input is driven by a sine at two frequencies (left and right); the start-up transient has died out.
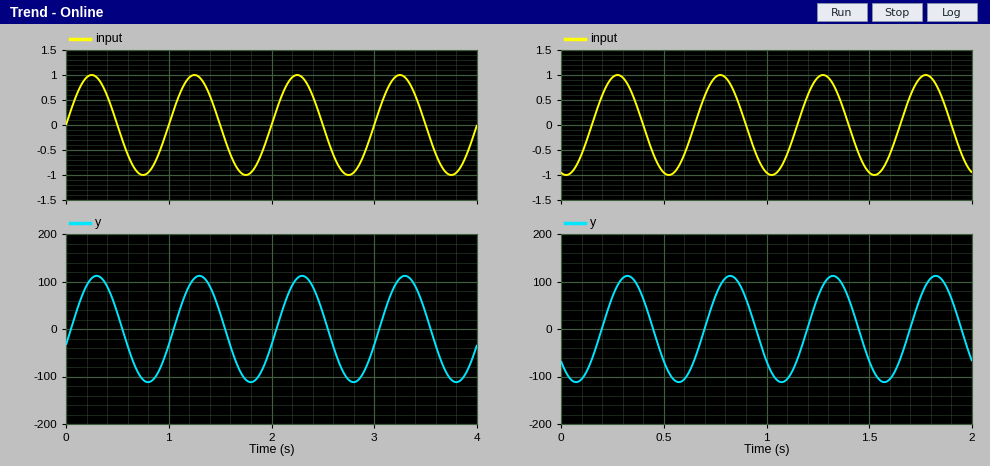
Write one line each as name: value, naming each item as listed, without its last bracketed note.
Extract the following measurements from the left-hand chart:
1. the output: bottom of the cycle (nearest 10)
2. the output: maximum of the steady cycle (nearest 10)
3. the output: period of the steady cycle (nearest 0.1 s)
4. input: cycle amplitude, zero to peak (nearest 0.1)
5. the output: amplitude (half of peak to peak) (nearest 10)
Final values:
the output: bottom of the cycle: -110
the output: maximum of the steady cycle: 110
the output: period of the steady cycle: 1.0 s
input: cycle amplitude, zero to peak: 1.0
the output: amplitude (half of peak to peak): 110
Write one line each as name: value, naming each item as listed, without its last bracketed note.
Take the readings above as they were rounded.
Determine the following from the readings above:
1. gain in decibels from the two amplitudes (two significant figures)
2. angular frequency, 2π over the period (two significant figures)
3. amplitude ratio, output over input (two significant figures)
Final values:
gain in decibels from the two amplitudes: 41 dB
angular frequency, 2π over the period: 6.3 rad/s
amplitude ratio, output over input: 110
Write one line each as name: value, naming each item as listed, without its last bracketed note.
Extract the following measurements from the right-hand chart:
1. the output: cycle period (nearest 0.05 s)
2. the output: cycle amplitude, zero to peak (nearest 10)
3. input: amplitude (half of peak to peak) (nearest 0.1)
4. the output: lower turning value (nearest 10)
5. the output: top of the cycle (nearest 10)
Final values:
the output: cycle period: 0.50 s
the output: cycle amplitude, zero to peak: 110
input: amplitude (half of peak to peak): 1.0
the output: lower turning value: -110
the output: top of the cycle: 110
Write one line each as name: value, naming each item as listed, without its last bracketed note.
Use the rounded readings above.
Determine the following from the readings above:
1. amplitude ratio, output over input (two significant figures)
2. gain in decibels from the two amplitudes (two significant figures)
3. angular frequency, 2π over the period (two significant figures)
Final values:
amplitude ratio, output over input: 110
gain in decibels from the two amplitudes: 41 dB
angular frequency, 2π over the period: 13 rad/s
